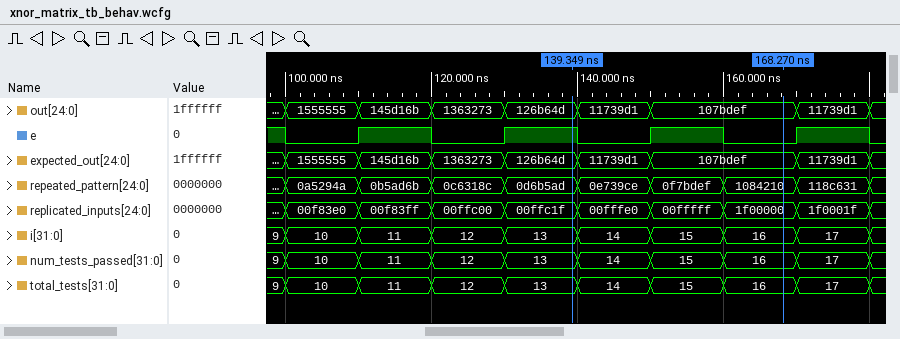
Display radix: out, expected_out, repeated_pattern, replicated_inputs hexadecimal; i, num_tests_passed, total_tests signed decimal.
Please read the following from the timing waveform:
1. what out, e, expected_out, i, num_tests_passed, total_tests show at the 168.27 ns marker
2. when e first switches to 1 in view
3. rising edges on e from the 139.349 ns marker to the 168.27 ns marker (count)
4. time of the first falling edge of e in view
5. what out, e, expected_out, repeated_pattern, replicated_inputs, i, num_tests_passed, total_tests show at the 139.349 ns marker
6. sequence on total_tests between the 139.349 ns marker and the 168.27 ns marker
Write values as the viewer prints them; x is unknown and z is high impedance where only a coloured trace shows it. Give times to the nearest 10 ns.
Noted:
out=107bdef, e=0, expected_out=107bdef, i=16, num_tests_passed=16, total_tests=16
110 ns
1
100 ns
out=126b64d, e=1, expected_out=126b64d, repeated_pattern=0d6b5ad, replicated_inputs=00ffc1f, i=13, num_tests_passed=13, total_tests=13
13, 14, 15, 16
